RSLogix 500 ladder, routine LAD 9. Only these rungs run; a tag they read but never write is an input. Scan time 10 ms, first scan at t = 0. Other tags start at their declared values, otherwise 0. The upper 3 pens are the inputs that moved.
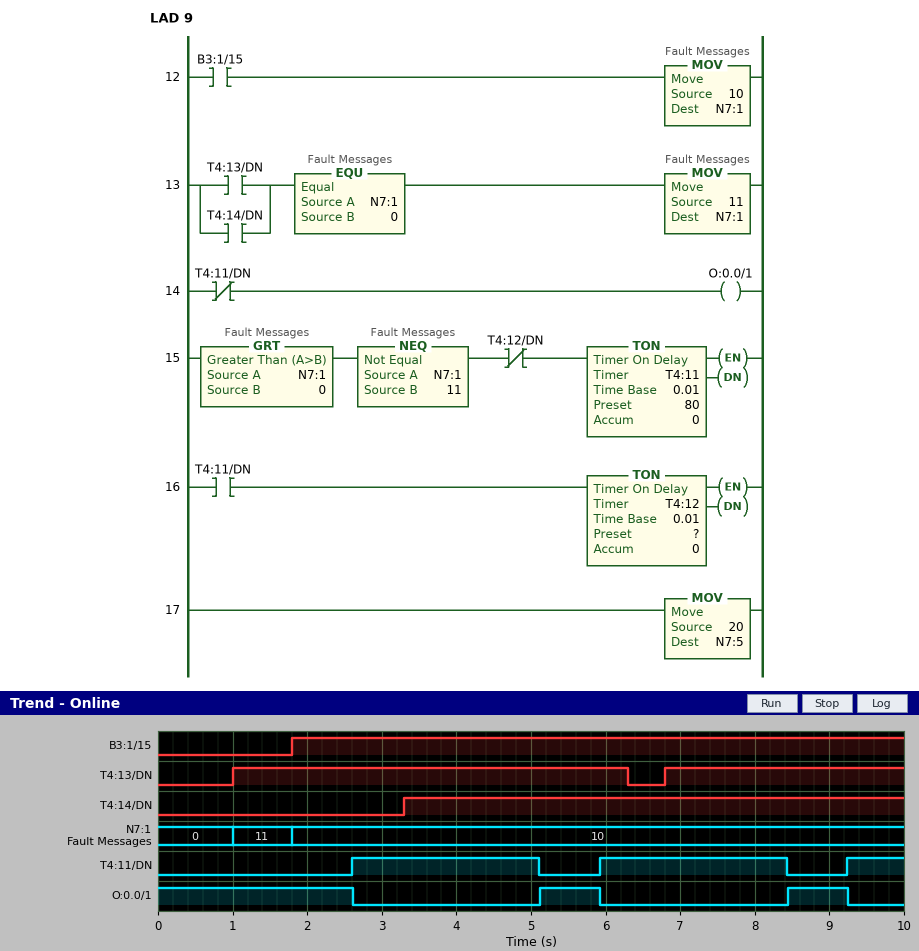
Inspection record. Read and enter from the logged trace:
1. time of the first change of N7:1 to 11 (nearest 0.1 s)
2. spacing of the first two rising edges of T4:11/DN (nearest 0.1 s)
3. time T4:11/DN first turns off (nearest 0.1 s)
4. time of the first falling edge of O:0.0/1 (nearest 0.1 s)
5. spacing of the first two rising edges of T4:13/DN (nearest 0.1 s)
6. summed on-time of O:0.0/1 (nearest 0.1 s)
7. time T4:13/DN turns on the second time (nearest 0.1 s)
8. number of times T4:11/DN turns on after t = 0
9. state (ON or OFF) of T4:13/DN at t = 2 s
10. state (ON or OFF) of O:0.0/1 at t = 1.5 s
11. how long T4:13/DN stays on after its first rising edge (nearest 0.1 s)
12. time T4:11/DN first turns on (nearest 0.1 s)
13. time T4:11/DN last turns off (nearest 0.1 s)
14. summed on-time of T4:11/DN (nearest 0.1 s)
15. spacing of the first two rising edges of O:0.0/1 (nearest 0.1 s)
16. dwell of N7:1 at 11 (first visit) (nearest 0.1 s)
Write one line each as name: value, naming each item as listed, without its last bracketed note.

time of the first change of N7:1 to 11: 1.0 s
spacing of the first two rising edges of T4:11/DN: 3.3 s
time T4:11/DN first turns off: 5.1 s
time of the first falling edge of O:0.0/1: 2.6 s
spacing of the first two rising edges of T4:13/DN: 5.8 s
summed on-time of O:0.0/1: 4.2 s
time T4:13/DN turns on the second time: 6.8 s
number of times T4:11/DN turns on after t = 0: 3
state (ON or OFF) of T4:13/DN at t = 2 s: ON
state (ON or OFF) of O:0.0/1 at t = 1.5 s: ON
how long T4:13/DN stays on after its first rising edge: 5.3 s
time T4:11/DN first turns on: 2.6 s
time T4:11/DN last turns off: 8.4 s
summed on-time of T4:11/DN: 5.8 s
spacing of the first two rising edges of O:0.0/1: 3.3 s
dwell of N7:1 at 11 (first visit): 0.8 s
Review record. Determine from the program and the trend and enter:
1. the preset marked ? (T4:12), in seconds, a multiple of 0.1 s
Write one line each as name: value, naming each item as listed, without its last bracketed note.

the preset marked ? (T4:12), in seconds, a multiple of 0.1 s: 2.5 s
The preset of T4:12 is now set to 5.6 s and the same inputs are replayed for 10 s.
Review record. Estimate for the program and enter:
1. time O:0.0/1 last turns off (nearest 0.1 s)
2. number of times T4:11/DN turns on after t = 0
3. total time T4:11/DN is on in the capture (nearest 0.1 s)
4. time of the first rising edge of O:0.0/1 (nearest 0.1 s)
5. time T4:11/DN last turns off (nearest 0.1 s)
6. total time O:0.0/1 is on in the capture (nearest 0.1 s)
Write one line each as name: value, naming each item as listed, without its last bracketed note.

time O:0.0/1 last turns off: 9.0 s
number of times T4:11/DN turns on after t = 0: 2
total time T4:11/DN is on in the capture: 6.6 s
time of the first rising edge of O:0.0/1: 8.2 s
time T4:11/DN last turns off: 8.2 s
total time O:0.0/1 is on in the capture: 3.4 s
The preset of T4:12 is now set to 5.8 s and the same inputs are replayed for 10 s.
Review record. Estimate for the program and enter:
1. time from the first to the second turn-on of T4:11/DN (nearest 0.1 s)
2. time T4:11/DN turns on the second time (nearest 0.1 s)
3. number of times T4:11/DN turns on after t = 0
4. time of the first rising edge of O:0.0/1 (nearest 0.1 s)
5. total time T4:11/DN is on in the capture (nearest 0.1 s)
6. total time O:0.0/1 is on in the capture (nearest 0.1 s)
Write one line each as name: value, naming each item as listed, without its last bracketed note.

time from the first to the second turn-on of T4:11/DN: 6.6 s
time T4:11/DN turns on the second time: 9.2 s
number of times T4:11/DN turns on after t = 0: 2
time of the first rising edge of O:0.0/1: 8.4 s
total time T4:11/DN is on in the capture: 6.6 s
total time O:0.0/1 is on in the capture: 3.4 s
